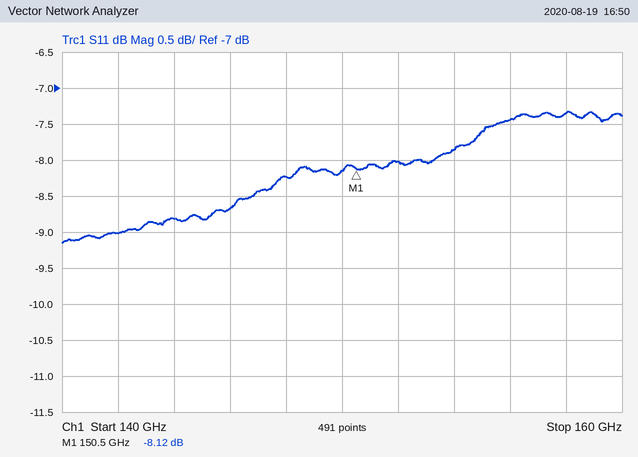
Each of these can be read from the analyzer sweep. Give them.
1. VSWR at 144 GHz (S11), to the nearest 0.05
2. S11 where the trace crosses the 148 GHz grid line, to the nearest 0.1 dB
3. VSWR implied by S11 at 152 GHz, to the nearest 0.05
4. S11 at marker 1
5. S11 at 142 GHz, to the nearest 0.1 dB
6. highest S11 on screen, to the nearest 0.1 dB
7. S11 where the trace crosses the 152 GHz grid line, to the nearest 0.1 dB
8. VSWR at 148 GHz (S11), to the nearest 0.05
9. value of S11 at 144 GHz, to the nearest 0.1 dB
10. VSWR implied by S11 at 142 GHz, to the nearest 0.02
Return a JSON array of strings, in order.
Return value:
["2.15", "-8.2 dB", "2.30", "-8.12 dB", "-9.0 dB", "-7.3 dB", "-8.0 dB", "2.25", "-8.8 dB", "2.10"]
